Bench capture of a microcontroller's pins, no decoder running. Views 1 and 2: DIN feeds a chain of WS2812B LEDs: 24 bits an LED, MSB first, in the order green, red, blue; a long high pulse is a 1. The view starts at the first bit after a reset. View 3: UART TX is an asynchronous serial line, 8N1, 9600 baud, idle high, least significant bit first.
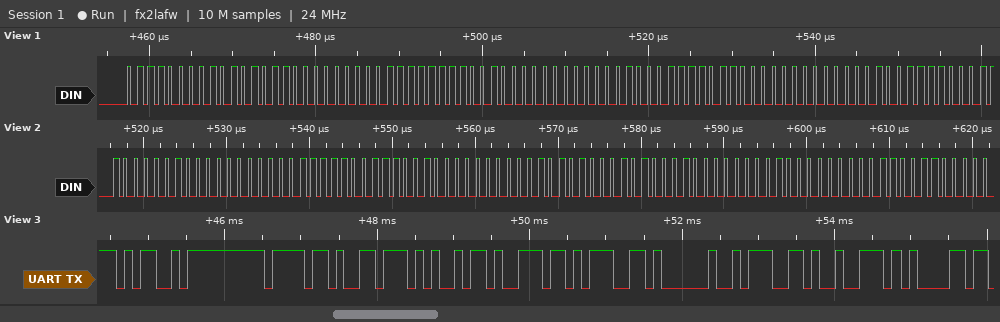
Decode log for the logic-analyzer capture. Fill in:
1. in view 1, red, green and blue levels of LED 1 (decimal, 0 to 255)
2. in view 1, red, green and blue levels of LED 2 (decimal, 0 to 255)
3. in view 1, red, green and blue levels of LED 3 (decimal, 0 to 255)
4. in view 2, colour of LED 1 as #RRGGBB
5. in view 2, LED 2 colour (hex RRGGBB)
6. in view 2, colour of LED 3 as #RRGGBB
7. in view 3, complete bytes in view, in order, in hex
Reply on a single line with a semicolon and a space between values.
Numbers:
171, 112, 0; 144, 127, 0; 96, 143, 0; #00823E; #007254; #005180; 4D 6F 76 69 6E 67 20 67 72 61
